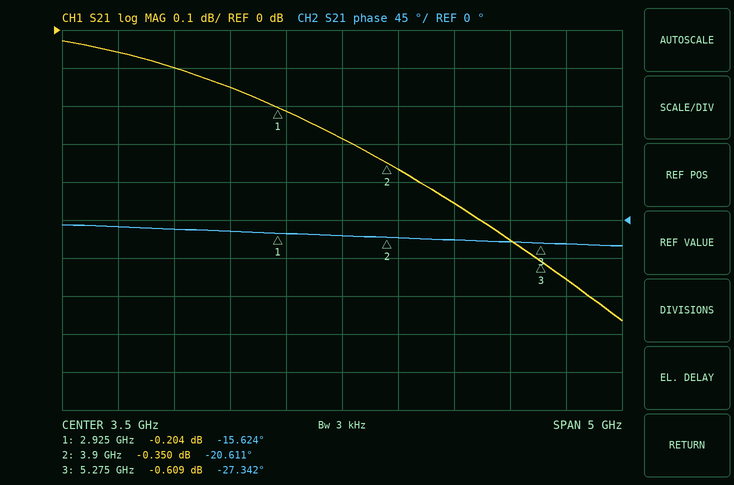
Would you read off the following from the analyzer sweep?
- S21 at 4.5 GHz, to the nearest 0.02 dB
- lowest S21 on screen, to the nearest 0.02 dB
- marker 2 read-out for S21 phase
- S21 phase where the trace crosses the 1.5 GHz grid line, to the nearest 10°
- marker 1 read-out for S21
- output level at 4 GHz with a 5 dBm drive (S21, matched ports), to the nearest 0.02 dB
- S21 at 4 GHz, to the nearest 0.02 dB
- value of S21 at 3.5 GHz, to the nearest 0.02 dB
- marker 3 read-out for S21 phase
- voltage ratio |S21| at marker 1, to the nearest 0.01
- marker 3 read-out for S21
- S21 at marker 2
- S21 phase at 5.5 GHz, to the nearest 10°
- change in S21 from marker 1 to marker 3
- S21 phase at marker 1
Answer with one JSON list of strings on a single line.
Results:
["-0.46 dB", "-0.76 dB", "-20.611°", "-10°", "-0.204 dB", "4.64 dBm", "-0.36 dB", "-0.28 dB", "-27.342°", "0.98", "-0.609 dB", "-0.350 dB", "-30°", "-0.405 dB", "-15.624°"]
